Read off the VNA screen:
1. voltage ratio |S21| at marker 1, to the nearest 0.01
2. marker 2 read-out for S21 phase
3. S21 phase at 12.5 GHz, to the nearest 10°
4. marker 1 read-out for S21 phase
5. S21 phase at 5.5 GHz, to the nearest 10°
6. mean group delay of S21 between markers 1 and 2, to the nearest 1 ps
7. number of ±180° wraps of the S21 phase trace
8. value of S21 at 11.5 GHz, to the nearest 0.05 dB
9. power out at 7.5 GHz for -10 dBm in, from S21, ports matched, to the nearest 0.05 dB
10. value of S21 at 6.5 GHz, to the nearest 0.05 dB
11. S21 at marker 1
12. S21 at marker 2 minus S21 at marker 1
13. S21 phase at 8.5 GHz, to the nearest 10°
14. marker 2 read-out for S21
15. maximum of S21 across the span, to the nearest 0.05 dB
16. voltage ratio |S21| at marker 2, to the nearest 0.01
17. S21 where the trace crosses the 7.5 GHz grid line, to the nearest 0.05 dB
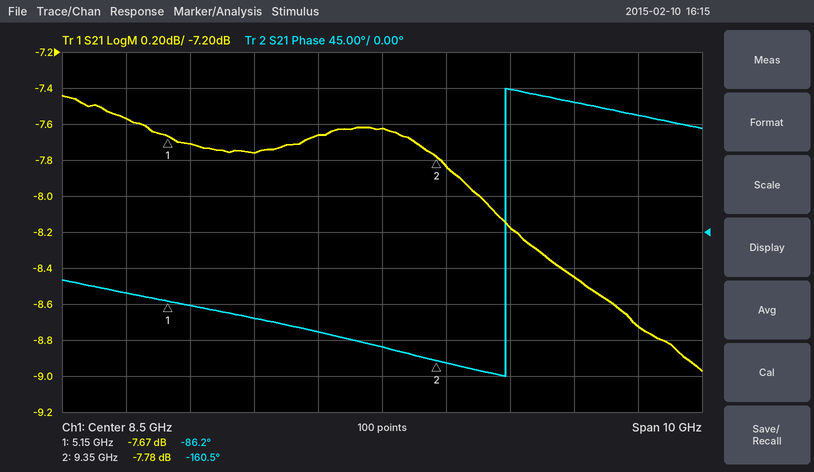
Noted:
0.41
-160.5°
150°
-86.2°
-90°
49 ps
1
-8.45 dB
-17.65 dBm
-7.75 dB
-7.67 dB
-0.11 dB
-140°
-7.78 dB
-7.45 dB
0.41
-7.65 dB
